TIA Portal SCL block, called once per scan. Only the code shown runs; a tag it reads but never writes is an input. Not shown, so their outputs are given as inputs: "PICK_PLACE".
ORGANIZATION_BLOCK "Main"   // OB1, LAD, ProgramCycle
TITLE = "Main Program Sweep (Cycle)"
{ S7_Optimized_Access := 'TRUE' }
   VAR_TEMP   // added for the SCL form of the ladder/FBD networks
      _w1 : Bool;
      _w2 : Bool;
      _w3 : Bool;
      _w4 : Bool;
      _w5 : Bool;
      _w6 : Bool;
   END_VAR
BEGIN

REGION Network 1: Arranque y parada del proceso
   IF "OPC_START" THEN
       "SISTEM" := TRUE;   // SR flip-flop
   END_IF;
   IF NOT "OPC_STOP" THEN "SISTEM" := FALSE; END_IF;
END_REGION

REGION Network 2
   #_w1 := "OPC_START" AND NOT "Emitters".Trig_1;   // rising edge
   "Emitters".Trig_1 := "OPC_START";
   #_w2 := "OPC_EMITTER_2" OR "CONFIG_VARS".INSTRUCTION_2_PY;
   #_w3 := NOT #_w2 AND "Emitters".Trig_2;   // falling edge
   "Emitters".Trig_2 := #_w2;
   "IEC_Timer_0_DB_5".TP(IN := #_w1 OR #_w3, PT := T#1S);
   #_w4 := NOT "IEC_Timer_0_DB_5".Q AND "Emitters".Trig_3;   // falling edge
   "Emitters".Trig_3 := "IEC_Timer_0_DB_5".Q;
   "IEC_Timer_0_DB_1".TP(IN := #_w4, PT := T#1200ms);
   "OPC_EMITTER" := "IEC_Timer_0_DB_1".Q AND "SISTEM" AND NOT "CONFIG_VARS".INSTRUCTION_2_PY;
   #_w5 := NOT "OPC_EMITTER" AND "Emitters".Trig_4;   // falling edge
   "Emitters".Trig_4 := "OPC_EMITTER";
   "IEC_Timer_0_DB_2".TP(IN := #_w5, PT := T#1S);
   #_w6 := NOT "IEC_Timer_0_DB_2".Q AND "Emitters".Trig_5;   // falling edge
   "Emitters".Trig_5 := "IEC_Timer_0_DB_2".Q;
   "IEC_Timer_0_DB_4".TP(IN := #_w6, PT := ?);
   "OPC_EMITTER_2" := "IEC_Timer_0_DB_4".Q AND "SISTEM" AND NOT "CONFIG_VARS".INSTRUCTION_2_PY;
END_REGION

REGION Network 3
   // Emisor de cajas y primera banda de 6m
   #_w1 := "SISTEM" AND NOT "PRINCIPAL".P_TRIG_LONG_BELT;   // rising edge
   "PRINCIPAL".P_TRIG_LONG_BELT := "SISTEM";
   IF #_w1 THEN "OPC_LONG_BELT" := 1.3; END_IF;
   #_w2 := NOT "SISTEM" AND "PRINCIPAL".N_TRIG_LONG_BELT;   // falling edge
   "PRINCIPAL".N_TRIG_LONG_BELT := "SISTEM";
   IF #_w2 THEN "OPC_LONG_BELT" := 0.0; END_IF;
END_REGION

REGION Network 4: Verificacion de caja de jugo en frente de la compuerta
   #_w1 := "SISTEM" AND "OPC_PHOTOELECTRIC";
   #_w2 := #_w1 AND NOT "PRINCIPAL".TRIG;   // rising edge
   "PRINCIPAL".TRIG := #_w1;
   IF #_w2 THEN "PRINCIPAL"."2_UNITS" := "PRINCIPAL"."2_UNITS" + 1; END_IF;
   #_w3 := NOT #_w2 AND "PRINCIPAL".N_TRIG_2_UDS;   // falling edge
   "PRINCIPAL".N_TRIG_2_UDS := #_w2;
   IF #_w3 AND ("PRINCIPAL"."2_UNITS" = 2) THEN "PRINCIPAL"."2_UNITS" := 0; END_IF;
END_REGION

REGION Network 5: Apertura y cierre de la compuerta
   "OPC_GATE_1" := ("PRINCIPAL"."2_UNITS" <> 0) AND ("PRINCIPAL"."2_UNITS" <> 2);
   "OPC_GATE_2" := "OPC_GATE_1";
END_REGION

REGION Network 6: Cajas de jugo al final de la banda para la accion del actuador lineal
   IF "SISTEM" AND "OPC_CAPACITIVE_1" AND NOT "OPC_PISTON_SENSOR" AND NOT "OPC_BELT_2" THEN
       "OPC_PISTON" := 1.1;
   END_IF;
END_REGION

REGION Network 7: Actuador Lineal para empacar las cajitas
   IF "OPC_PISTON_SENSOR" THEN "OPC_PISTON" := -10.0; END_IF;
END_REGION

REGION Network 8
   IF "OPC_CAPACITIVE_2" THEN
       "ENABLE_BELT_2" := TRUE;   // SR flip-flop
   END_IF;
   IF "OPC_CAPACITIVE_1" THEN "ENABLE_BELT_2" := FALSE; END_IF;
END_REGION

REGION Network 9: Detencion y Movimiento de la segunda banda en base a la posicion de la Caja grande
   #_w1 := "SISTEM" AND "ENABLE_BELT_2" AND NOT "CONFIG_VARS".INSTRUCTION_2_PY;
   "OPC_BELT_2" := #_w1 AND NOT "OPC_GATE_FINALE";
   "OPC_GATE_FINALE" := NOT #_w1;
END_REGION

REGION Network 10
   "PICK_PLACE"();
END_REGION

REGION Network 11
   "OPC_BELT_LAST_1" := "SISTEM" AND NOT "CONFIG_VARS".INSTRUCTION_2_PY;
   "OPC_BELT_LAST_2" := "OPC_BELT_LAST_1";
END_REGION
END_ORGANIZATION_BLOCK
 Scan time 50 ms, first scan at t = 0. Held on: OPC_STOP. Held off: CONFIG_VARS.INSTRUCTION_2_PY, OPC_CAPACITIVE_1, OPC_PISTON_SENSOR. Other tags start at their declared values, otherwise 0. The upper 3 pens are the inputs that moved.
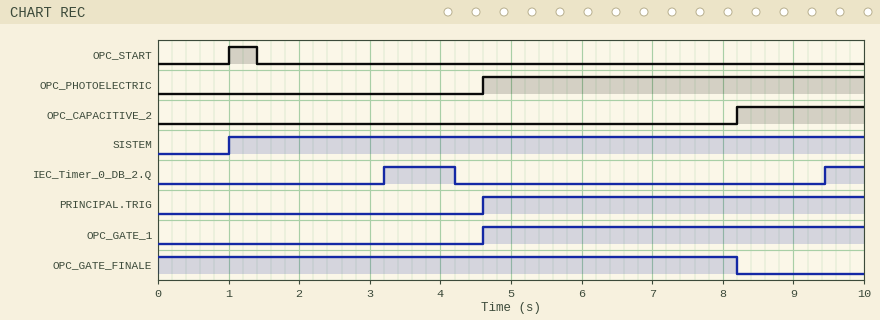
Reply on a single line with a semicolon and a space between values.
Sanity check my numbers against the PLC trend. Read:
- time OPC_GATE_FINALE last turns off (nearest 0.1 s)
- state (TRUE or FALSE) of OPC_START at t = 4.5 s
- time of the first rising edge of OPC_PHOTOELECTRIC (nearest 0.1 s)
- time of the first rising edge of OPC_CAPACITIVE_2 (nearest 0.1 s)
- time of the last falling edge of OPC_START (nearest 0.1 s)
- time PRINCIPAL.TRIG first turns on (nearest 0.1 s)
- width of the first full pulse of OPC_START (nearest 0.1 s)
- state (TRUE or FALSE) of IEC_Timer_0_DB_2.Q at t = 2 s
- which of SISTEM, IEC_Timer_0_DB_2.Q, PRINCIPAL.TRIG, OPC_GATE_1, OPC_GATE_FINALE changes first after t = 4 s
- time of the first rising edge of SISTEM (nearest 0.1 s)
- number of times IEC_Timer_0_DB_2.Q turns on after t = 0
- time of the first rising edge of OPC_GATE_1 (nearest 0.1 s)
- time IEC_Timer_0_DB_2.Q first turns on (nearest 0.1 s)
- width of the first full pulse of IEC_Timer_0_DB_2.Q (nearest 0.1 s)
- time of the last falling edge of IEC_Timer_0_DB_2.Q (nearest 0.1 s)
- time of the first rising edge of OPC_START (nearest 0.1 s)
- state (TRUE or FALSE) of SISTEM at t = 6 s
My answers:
8.2 s; FALSE; 4.6 s; 8.2 s; 1.4 s; 4.6 s; 0.4 s; FALSE; IEC_Timer_0_DB_2.Q; 1.0 s; 2; 4.6 s; 3.2 s; 1.0 s; 4.2 s; 1.0 s; TRUE
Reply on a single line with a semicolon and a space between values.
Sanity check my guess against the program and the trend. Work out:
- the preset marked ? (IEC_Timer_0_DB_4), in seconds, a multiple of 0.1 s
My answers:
3.0 s
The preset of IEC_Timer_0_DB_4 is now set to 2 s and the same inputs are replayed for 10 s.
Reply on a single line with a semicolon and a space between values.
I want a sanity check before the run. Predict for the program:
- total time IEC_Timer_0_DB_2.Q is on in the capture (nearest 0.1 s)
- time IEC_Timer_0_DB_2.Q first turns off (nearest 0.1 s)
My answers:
2.0 s; 4.2 s
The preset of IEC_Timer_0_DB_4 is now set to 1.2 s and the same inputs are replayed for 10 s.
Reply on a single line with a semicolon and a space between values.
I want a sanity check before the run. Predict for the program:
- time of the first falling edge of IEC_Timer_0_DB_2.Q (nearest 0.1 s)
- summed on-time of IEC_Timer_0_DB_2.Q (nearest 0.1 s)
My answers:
4.2 s; 2.0 s
